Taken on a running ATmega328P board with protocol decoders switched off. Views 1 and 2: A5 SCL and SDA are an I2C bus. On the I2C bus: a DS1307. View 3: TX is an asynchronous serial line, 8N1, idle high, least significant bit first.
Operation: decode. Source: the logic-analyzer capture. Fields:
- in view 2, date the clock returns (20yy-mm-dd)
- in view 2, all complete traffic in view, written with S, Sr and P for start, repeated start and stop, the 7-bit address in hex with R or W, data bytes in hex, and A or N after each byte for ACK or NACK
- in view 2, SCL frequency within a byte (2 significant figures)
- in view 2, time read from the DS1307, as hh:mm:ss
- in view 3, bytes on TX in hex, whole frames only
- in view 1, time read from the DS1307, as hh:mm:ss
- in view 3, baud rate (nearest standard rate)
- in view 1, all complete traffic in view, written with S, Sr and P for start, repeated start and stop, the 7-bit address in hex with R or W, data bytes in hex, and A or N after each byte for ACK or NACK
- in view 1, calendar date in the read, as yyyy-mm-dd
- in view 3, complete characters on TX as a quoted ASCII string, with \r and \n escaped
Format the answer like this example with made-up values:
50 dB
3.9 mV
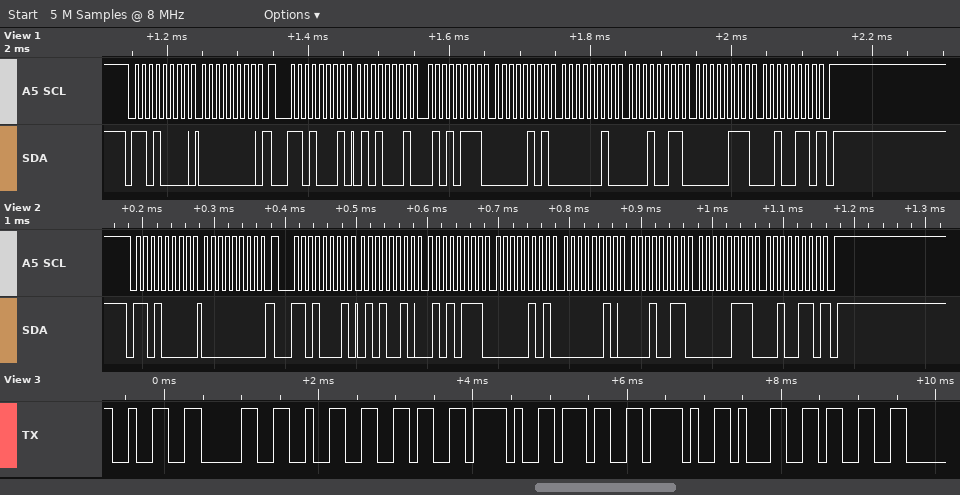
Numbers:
2026-07-13
S 68W A 00 A Sr 68R A 52 A 57 A 05 A 02 A 13 A 07 A 26 N P
100 kHz
05:57:52
32 30 32 36 2F 37 2F 31 33
05:57:51
9600 baud
S 68W A 00 A Sr 68R A 51 A 57 A 05 A 02 A 13 A 07 A 26 N P
2026-07-13
"2026/7/13"
